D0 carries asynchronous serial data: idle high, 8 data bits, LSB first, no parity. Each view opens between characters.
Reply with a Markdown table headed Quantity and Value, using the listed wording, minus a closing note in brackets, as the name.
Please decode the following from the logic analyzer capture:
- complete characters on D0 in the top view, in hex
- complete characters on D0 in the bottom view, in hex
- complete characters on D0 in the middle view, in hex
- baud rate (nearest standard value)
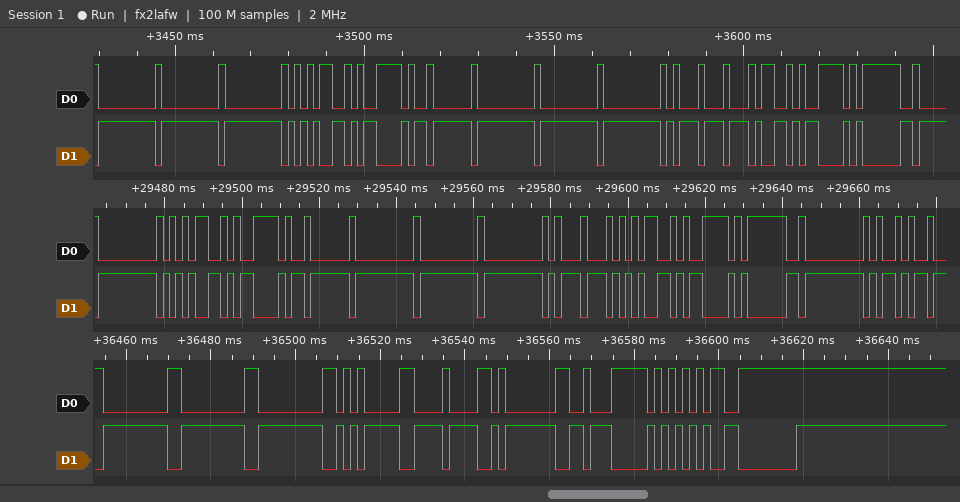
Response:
| Quantity | Value |
|---|---|
| complete characters on D0 in the top view, in hex | 00, 00, 00, 35, 79, 02, 00, 00, 00, 11, 34, 79, 3F |
| complete characters on D0 in the bottom view, in hex | 00, 00, 00, 05, 08, 01, E2, 55, FE |
| complete characters on D0 in the middle view, in hex | 00, 35, 79, 02, 00, 00, 00, 11, 35, 79, 3F, 00, 29 |
| baud rate | 600 baud |
